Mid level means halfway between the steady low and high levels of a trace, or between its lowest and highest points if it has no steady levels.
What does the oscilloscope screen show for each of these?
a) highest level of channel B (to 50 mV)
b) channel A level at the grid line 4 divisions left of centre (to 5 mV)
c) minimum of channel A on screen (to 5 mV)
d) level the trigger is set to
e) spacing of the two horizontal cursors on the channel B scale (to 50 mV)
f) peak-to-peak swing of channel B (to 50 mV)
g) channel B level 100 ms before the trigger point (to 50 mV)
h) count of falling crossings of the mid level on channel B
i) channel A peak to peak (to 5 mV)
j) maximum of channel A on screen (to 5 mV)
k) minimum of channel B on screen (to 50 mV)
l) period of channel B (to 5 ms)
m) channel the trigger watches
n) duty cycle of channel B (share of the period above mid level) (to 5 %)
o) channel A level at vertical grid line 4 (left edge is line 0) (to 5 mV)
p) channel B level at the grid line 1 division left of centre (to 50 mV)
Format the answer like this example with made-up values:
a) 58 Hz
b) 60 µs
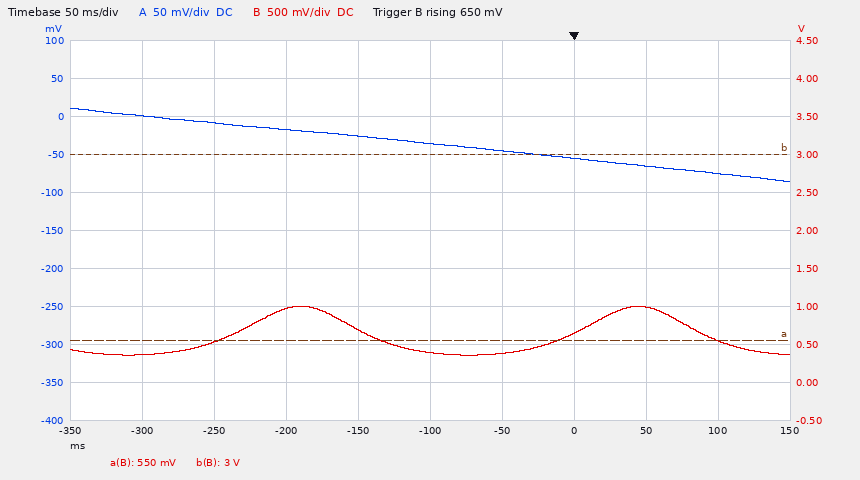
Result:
a) 1.00 V
b) 0 mV
c) -85 mV
d) 650 mV
e) 2.45 V
f) 650 mV
g) 400 mV
h) 2
i) 95 mV
j) 10 mV
k) 350 mV
l) 235 ms
m) channel B
n) 35 %
o) -25 mV
p) 700 mV
